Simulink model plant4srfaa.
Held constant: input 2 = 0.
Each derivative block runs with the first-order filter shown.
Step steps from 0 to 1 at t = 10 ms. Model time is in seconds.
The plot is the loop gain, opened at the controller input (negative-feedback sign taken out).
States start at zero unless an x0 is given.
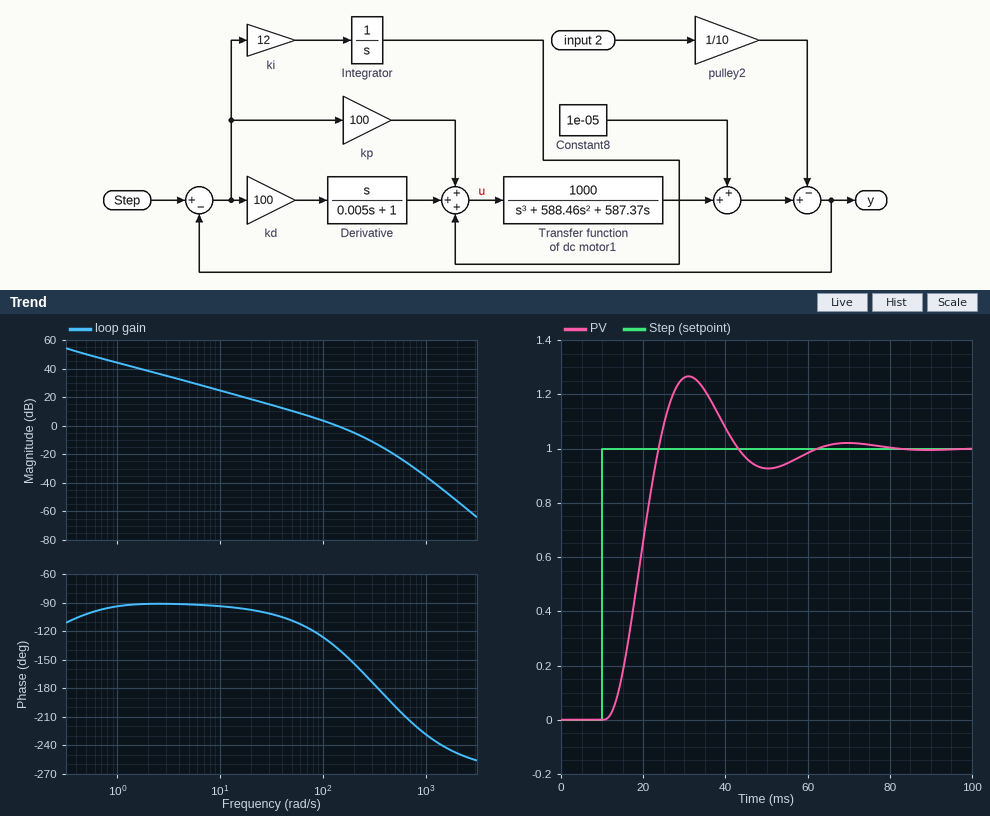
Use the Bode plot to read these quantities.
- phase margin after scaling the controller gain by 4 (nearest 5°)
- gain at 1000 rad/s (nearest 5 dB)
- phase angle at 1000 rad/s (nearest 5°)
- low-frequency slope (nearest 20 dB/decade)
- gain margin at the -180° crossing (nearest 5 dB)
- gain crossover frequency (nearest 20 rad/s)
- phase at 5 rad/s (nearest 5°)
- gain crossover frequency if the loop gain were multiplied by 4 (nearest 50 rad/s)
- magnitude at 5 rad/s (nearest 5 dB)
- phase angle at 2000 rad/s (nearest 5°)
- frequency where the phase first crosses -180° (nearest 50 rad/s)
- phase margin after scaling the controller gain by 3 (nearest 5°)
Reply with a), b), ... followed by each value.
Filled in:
a) 5°
b) -35 dB
c) -230°
d) -20 dB/decade
e) 15 dB
f) 140 rad/s
g) -90°
h) 300 rad/s
i) 30 dB
j) -250°
k) 350 rad/s
l) 10°
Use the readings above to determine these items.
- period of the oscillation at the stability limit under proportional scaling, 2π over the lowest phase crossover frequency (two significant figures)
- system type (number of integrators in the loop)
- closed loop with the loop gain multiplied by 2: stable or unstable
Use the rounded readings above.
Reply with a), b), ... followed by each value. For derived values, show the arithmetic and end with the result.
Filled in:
a) 2π / 350 = 0.018 s
b) 1
c) stable
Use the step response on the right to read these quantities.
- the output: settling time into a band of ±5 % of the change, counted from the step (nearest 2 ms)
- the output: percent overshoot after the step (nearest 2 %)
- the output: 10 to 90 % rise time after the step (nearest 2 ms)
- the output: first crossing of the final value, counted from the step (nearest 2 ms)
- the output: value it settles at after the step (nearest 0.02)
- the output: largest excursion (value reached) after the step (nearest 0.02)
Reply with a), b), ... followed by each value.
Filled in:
a) 46 ms
b) 26 %
c) 8 ms
d) 14 ms
e) 1.00
f) 1.26
